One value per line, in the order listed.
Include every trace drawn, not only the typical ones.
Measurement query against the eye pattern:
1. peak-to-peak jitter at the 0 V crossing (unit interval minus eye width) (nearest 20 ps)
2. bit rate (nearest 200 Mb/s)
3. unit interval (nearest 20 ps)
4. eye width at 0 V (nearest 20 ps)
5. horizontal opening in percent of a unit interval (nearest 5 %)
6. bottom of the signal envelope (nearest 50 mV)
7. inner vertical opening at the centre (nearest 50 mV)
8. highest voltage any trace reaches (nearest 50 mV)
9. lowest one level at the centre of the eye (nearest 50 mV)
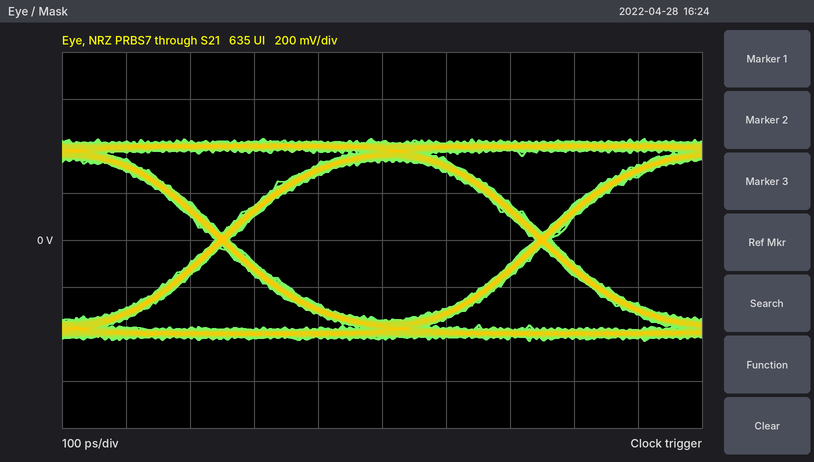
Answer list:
20 ps
2.0 Gb/s
500 ps
480 ps
95 %
-450 mV
700 mV
450 mV
350 mV
